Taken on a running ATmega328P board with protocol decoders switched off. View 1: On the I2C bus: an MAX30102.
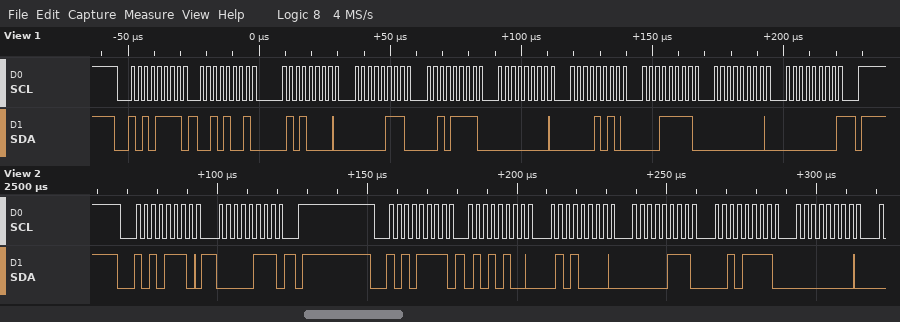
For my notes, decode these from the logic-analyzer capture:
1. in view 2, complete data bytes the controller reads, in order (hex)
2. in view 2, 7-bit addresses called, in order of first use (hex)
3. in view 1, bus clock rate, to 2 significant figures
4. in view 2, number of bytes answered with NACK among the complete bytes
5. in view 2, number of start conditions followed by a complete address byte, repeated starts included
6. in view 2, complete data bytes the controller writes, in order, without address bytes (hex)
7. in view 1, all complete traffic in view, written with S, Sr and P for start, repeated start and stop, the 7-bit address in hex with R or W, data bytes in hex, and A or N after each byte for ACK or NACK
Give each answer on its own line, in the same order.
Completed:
54 50 07 2F 00
0x57
400 kHz
0
2
07
S 57R A 29 A 50 A 07 A 2F A 00 A 0A A 1F A 00 A 00 N P
